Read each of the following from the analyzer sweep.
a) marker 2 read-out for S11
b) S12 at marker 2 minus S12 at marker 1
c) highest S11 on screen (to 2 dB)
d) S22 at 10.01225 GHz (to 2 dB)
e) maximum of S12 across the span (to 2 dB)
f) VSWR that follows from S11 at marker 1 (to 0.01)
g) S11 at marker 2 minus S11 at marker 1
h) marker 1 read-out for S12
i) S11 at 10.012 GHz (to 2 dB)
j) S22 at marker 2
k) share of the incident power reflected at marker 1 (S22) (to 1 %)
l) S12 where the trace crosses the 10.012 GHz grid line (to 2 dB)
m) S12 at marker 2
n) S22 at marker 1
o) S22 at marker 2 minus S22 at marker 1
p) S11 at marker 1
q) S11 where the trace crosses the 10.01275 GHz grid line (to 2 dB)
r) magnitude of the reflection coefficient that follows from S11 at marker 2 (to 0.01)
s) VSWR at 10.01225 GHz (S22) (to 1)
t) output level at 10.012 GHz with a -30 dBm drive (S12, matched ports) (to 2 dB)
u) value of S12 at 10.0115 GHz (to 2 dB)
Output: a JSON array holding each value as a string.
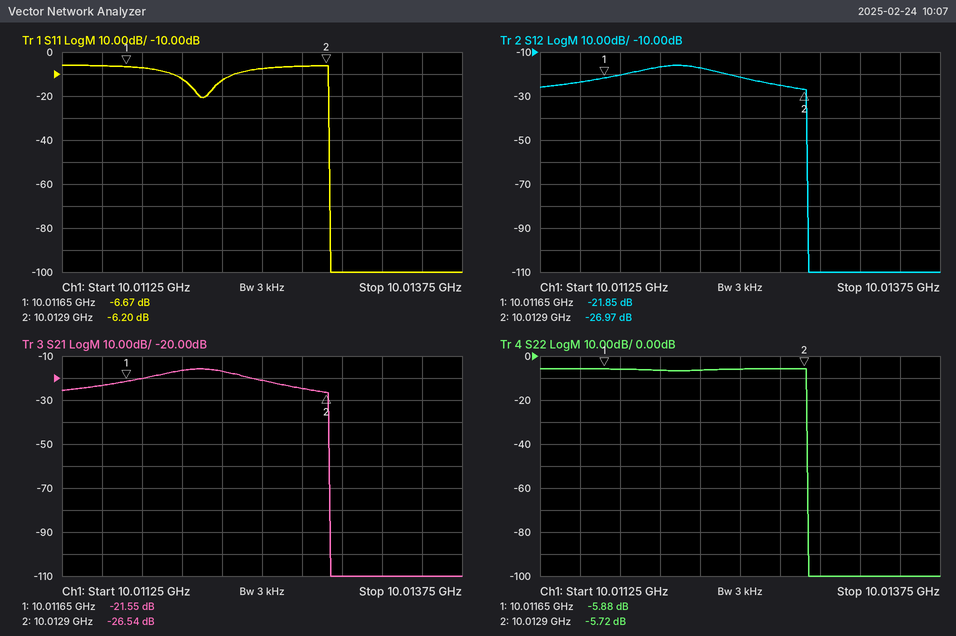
["-6.20 dB", "-5.12 dB", "-6 dB", "-6 dB", "-16 dB", "2.73", "0.47 dB", "-21.85 dB", "-12 dB", "-5.72 dB", "26 %", "-16 dB", "-26.97 dB", "-5.88 dB", "0.16 dB", "-6.67 dB", "-6 dB", "0.49", "3", "-46 dBm", "-24 dB"]
